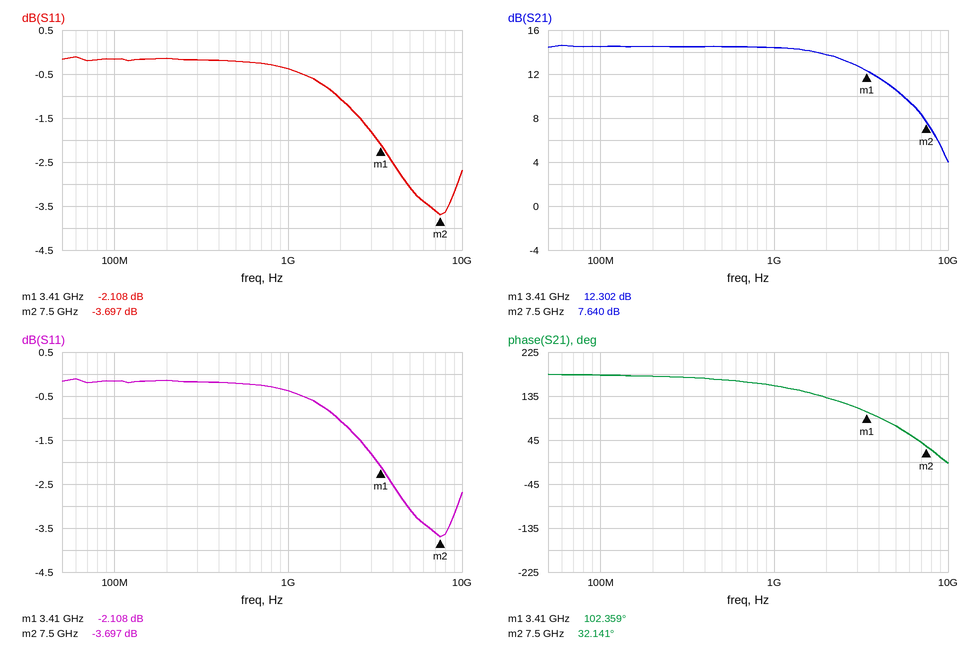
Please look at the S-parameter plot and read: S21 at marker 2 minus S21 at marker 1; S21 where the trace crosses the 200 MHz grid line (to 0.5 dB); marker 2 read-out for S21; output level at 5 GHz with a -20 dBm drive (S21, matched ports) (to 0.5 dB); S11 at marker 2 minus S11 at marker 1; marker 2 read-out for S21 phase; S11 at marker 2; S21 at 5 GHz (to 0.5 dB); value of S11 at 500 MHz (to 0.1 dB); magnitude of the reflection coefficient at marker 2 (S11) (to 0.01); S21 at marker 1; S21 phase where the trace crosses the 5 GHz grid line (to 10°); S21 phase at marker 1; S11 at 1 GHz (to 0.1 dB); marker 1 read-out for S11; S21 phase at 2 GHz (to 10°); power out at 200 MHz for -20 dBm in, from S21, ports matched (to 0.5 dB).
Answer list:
-4.662 dB
14.5 dB
7.640 dB
-9.5 dBm
-1.589 dB
32.141°
-3.697 dB
10.5 dB
-0.2 dB
0.65
12.302 dB
70°
102.359°
-0.4 dB
-2.108 dB
130°
-5.5 dBm
